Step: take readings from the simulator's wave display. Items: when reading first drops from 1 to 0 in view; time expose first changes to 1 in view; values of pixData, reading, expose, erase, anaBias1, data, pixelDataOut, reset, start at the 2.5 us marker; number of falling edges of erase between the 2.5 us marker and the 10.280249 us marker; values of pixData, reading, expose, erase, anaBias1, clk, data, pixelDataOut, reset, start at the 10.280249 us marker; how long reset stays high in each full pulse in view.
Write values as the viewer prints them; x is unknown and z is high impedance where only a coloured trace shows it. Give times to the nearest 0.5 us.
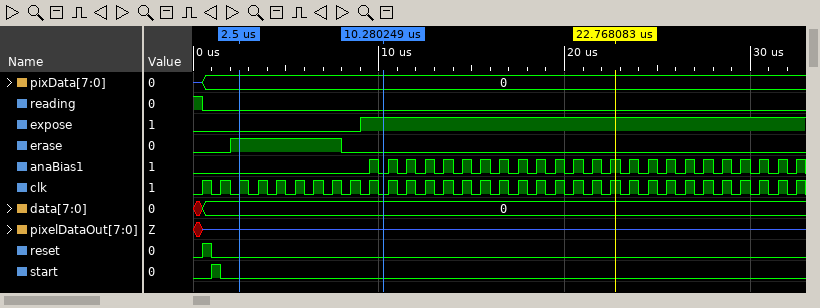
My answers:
0.5 us
9 us
pixData=0, reading=0, expose=0, erase=1, anaBias1=0, data=0, pixelDataOut=z, reset=0, start=0
1
pixData=0, reading=0, expose=1, erase=0, anaBias1=0, clk=0, data=0, pixelDataOut=z, reset=0, start=0
0.5 us
